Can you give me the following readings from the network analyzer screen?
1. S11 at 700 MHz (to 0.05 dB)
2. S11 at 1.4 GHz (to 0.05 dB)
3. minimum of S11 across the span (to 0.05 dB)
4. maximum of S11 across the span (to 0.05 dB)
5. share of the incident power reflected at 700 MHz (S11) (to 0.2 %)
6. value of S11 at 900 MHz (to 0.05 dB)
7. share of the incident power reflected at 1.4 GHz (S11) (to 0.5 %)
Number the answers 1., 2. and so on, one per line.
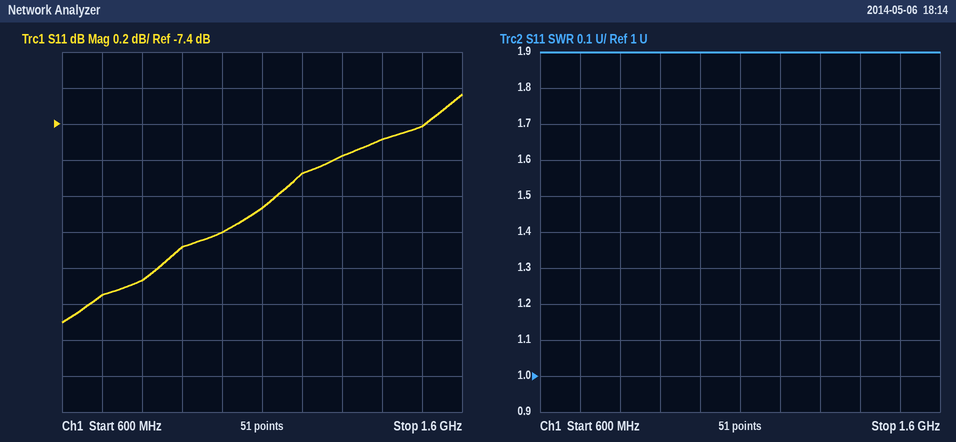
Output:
1. -8.35 dB
2. -7.50 dB
3. -8.50 dB
4. -7.25 dB
5. 14.6 %
6. -8.10 dB
7. 18.0 %
